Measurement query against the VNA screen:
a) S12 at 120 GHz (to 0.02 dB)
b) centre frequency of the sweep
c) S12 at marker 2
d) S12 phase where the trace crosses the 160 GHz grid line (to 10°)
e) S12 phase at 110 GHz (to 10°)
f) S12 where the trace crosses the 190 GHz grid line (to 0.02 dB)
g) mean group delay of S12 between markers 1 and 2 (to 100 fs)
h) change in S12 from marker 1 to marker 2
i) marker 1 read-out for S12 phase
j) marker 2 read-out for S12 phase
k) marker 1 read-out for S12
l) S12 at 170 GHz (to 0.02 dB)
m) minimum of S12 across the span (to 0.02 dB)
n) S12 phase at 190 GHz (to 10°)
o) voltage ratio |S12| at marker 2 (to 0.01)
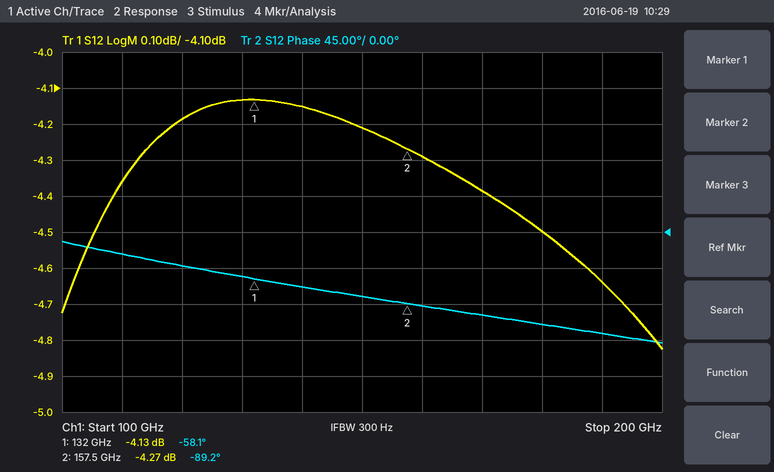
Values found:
-4.18 dB
150 GHz
-4.27 dB
-90°
-30°
-4.64 dB
3.4 ps
-0.14 dB
-58.1°
-89.2°
-4.13 dB
-4.38 dB
-4.82 dB
-130°
0.61
